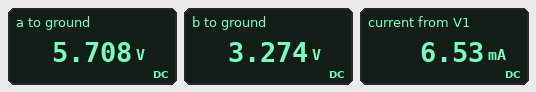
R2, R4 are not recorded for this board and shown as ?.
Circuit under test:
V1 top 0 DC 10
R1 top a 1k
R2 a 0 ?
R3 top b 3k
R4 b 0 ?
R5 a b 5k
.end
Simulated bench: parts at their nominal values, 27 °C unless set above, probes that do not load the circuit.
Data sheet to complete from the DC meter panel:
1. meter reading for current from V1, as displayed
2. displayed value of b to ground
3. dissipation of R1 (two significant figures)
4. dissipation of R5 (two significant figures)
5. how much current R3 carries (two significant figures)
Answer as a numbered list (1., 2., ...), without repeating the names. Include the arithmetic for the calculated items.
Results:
1. 6.53 mA
2. 3.274 V
3. (10 V - 5.708 V)^2 / 1 kΩ = 18 mW
4. (5.708 V - 3.274 V)^2 / 5 kΩ = 1.2 mW
5. (10 V - 3.274 V) / 3 kΩ = 2.2 mA
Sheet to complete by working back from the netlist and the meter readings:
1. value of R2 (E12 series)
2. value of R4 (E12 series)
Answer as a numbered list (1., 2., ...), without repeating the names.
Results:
1. 1.5 kΩ
2. 1.2 kΩ
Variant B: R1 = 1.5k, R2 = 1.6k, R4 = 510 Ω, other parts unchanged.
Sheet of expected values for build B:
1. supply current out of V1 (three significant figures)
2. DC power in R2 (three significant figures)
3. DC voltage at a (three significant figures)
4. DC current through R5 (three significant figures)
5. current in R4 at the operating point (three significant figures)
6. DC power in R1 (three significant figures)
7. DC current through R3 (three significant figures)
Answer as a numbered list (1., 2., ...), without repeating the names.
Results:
1. 6.30 mA
2. 13.8 mW
3. 4.70 V
4. 597 µA
5. 3.36 mA
6. 18.7 mW
7. 2.76 mA
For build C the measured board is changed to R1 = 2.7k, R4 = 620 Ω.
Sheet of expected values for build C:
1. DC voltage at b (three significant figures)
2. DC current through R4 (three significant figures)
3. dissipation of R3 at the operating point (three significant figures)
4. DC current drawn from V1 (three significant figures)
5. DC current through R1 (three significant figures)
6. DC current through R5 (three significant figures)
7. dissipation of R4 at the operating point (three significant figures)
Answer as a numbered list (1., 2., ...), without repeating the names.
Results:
1. 1.86 V
2. 3.00 mA
3. 22.1 mW
4. 5.20 mA
5. 2.48 mA
6. 287 µA
7. 5.58 mW
